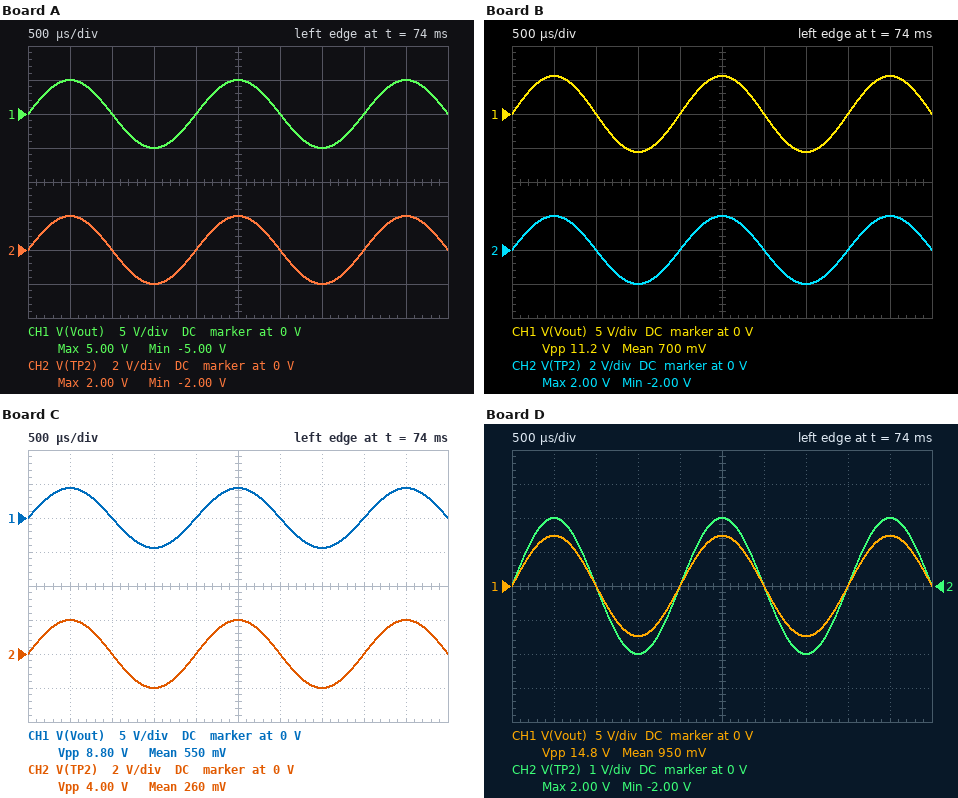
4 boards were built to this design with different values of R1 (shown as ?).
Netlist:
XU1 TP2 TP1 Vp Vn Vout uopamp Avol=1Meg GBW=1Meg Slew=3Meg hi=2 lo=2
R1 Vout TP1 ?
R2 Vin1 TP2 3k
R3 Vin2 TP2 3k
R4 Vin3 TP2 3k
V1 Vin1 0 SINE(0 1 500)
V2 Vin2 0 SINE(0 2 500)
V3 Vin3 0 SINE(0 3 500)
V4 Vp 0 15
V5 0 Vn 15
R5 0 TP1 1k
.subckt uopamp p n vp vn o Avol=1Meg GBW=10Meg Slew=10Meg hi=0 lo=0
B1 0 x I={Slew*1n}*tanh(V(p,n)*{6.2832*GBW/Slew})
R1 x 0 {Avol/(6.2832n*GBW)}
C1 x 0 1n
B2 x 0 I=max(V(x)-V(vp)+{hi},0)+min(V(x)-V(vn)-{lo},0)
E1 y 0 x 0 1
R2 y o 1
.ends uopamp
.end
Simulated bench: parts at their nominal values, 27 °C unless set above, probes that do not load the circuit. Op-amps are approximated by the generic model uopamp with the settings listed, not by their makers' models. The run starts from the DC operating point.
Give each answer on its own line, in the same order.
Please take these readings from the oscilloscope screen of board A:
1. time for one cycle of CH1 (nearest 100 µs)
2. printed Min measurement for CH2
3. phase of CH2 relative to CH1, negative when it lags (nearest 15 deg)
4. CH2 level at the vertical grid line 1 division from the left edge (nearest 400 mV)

2.0 ms
-2.00 V
0 deg
2.0 V
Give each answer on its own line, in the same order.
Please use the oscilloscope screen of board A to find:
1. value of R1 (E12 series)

1.5 kΩ
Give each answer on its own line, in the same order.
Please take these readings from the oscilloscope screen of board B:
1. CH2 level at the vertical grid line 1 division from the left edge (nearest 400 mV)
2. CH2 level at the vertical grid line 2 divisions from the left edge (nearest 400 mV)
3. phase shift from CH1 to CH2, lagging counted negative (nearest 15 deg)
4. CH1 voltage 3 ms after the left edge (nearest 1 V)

2.0 V
0 V
0 deg
0 V
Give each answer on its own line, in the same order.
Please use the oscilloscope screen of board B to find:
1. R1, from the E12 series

1.8 kΩ
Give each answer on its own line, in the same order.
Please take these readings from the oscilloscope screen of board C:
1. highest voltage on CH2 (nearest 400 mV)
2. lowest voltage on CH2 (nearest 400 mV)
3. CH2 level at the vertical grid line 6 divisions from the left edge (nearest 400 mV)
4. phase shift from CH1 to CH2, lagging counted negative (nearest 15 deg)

2.0 V
-2.0 V
0 V
0 deg
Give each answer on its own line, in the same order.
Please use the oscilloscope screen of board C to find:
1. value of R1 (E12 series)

1.2 kΩ
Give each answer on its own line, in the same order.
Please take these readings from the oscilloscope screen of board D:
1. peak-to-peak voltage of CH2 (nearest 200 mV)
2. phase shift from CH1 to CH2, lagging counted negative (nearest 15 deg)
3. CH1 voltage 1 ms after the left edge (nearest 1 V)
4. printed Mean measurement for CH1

4.0 V
0 deg
0 V
950 mV
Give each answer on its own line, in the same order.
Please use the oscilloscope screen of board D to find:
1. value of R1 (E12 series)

2.7 kΩ
